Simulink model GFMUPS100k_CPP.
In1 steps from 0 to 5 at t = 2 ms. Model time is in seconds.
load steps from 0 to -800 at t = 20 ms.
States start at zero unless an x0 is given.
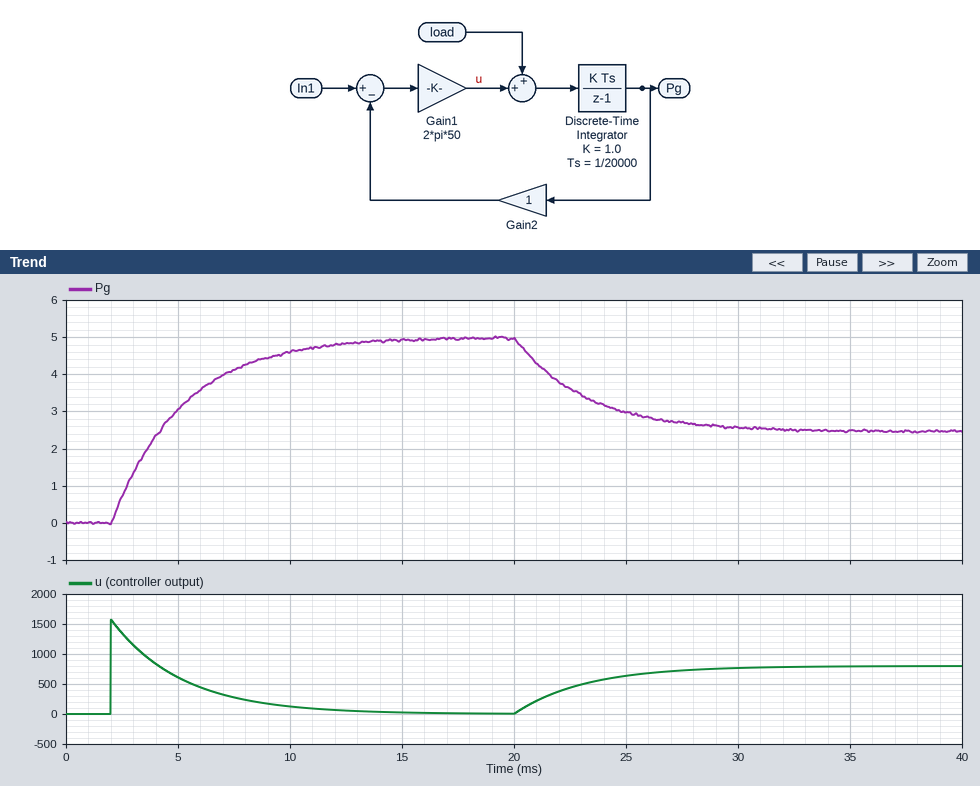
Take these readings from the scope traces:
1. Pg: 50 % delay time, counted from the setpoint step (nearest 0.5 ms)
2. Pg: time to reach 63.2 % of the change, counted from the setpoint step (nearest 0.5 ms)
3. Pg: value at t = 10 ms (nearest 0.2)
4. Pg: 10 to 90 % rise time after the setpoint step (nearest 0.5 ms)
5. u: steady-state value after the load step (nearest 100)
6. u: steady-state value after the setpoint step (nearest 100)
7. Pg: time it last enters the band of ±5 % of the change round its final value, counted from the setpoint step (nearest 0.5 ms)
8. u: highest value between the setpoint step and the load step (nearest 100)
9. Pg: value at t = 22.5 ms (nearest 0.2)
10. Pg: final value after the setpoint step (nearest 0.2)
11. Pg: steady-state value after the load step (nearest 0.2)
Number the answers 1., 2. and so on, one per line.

1. 2.0 ms
2. 3.0 ms
3. 4.6
4. 7.0 ms
5. 800
6. 0
7. 9.5 ms
8. 1600
9. 3.6
10. 5.0
11. 2.4
